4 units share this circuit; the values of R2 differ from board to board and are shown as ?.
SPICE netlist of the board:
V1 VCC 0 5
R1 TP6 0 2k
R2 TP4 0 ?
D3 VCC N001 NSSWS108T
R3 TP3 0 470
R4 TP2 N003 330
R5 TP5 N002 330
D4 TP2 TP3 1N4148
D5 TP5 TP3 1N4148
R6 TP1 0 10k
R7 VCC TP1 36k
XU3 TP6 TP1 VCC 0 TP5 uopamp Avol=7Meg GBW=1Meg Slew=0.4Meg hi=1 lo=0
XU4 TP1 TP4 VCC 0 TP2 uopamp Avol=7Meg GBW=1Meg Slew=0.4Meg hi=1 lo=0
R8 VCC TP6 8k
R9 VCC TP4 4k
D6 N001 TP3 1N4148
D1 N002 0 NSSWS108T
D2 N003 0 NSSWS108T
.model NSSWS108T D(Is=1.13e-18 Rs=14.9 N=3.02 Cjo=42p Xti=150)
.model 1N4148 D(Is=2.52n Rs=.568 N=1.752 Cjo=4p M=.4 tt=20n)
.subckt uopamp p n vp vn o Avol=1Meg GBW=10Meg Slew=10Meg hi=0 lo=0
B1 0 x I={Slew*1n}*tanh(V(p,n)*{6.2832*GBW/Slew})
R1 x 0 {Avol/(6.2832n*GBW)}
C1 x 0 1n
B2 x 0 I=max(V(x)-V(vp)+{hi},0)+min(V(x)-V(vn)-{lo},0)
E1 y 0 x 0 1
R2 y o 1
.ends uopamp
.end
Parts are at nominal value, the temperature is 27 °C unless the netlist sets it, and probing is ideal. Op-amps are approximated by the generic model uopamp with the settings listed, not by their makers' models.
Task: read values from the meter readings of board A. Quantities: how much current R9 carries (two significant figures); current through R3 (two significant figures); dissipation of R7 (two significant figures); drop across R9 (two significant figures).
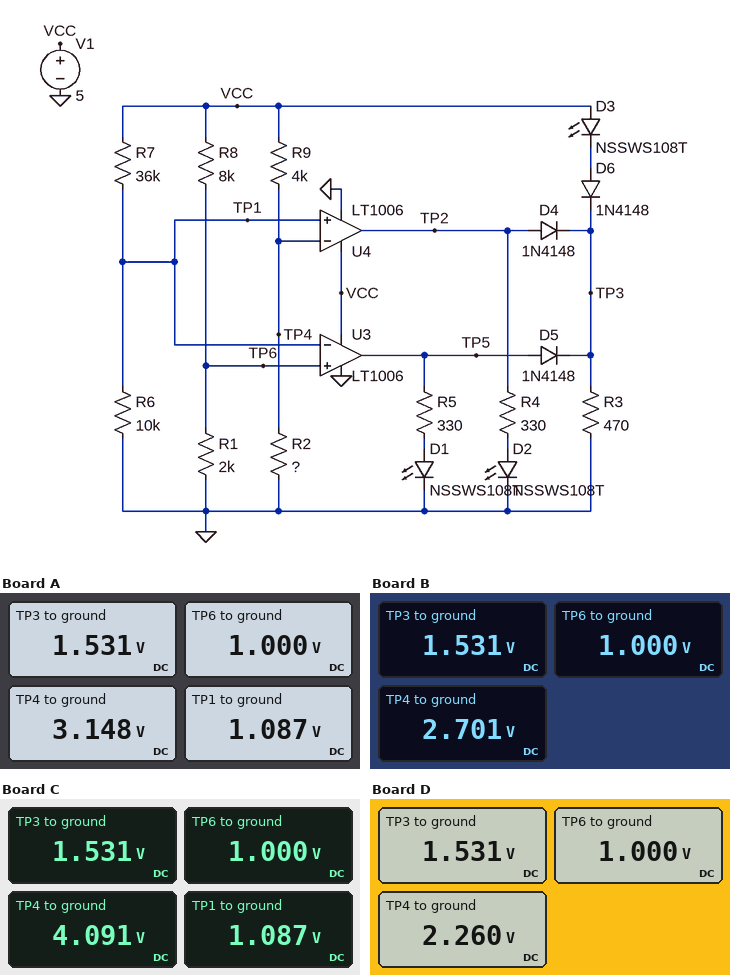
460 µA
3.3 mA
430 µW
1.9 V
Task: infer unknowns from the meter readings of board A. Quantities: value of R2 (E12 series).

6.8 kΩ
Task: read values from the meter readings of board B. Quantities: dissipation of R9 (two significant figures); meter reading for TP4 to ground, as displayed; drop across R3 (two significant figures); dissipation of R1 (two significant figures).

1.3 mW
2.701 V
1.5 V
500 µW
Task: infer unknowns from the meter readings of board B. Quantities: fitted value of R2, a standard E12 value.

4.7 kΩ
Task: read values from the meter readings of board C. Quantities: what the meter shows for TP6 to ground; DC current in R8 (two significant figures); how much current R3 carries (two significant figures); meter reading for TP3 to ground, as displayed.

1.000 V
500 µA
3.3 mA
1.531 V
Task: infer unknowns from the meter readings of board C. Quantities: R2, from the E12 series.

18 kΩ
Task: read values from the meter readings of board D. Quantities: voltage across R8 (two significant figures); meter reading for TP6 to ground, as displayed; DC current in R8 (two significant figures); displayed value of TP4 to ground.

4.0 V
1.000 V
500 µA
2.260 V
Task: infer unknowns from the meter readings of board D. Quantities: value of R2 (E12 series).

3.3 kΩ
